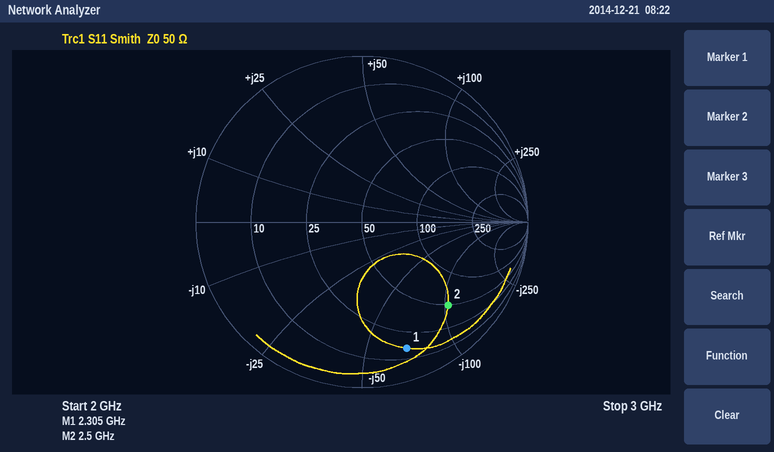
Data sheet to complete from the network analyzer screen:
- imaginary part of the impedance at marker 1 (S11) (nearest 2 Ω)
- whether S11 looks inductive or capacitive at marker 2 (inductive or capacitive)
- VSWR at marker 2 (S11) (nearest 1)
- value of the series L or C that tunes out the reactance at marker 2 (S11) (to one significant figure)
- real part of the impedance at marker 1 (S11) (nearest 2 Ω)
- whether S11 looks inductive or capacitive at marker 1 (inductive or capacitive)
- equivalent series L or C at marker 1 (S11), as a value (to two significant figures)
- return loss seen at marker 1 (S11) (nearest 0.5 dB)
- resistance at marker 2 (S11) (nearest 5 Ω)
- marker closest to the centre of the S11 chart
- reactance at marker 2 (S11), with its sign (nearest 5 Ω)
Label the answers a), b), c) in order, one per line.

a) -68 Ω
b) capacitive
c) 6
d) 7 nH
e) 16 Ω
f) capacitive
g) 1.0 pF
h) 2.0 dB
i) 50 Ω
j) marker 2
k) -105 Ω
